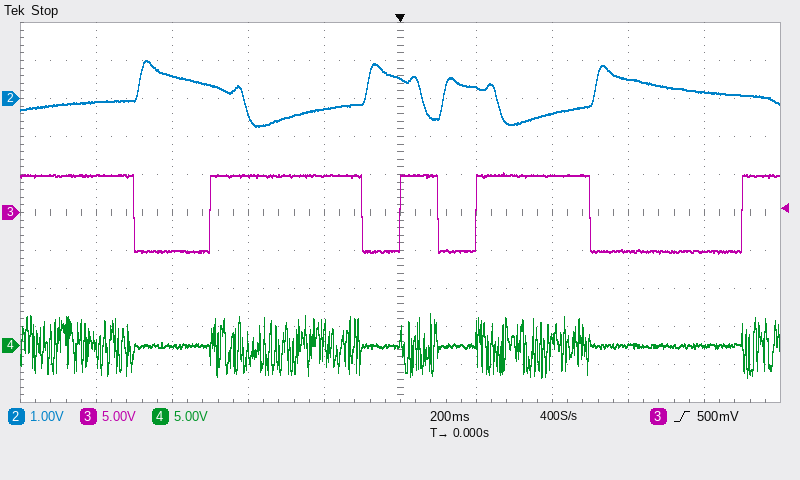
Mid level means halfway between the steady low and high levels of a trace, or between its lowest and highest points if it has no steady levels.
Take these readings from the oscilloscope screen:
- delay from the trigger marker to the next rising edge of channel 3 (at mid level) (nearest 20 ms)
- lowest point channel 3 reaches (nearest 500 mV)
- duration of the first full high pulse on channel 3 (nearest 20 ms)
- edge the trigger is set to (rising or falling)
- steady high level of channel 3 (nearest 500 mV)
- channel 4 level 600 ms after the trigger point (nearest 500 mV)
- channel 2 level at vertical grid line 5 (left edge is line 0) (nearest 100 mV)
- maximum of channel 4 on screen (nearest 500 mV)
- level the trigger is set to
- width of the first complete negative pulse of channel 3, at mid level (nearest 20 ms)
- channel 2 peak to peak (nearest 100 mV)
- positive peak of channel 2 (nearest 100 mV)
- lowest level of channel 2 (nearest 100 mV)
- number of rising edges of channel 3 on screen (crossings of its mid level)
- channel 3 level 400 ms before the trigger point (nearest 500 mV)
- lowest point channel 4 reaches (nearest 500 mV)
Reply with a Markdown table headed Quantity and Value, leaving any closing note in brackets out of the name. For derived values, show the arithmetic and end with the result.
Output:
| Quantity | Value |
|---|---|
| delay from the trigger marker to the next rising edge of channel 3 (at mid level) | 200 ms |
| lowest point channel 3 reaches | -5.5 V |
| duration of the first full high pulse on channel 3 | 400 ms |
| edge the trigger is set to | rising |
| steady high level of channel 3 | 5.0 V |
| channel 4 level 600 ms after the trigger point | 0.0 V |
| channel 2 level at vertical grid line 5 (left edge is line 0) | 500 mV |
| maximum of channel 4 on screen | 4.0 V |
| level the trigger is set to | 500 mV |
| width of the first complete negative pulse of channel 3, at mid level | 200 ms |
| channel 2 peak to peak | 1.0 V − (-700 mV) = 1.7 V |
| positive peak of channel 2 | 1.0 V |
| lowest level of channel 2 | -700 mV |
| number of rising edges of channel 3 on screen | 4 |
| channel 3 level 400 ms before the trigger point | 5.0 V |
| lowest point channel 4 reaches | -4.0 V |
